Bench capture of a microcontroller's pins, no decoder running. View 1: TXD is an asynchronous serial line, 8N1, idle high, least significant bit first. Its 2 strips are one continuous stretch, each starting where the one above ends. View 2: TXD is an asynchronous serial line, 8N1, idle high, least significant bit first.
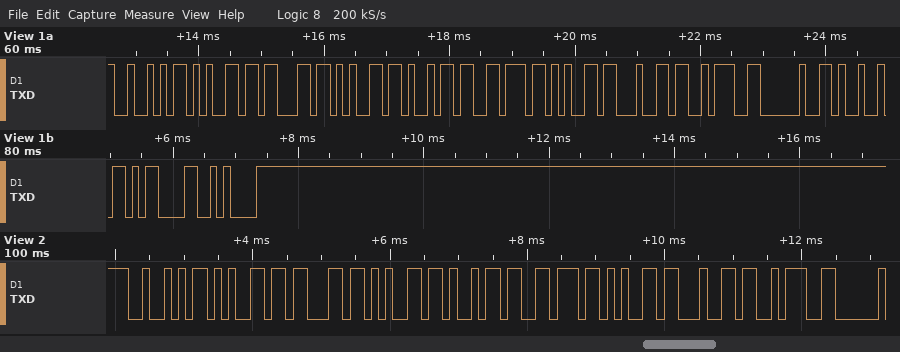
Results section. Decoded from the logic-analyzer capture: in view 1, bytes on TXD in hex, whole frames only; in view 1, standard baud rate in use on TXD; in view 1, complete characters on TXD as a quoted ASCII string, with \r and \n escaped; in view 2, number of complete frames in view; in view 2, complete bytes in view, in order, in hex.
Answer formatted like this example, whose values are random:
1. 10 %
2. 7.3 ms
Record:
1. 0x52 0x65 0x63 0x65 0x69 0x76 0x65 0x64 0x3A 0x20 0x49 0x0D 0x0A
2. 9600 baud
3. "Received: I\r\n"
4. 9
5. 52 65 63 65 69 76 65 64 3A
